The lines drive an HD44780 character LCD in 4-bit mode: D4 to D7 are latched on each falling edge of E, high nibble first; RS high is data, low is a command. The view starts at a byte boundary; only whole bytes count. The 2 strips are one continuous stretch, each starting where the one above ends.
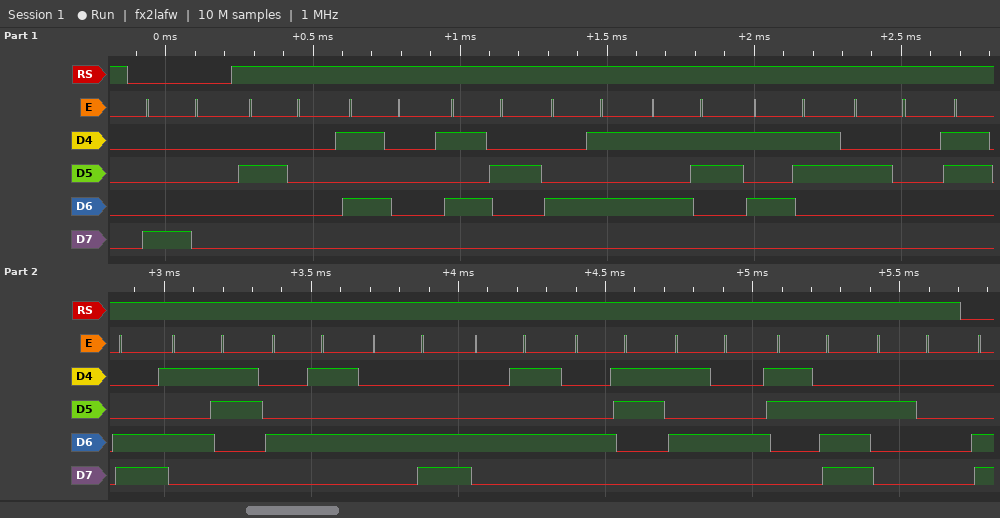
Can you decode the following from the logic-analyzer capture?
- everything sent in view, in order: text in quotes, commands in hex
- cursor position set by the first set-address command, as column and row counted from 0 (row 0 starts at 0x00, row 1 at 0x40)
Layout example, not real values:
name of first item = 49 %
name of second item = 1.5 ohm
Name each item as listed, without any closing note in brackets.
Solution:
everything sent in view, in order: text in quotes, commands in hex = 0x80 " PRESS <SELECT> "
cursor position set by the first set-address command, as column and row counted from 0 = column 0, row 0
